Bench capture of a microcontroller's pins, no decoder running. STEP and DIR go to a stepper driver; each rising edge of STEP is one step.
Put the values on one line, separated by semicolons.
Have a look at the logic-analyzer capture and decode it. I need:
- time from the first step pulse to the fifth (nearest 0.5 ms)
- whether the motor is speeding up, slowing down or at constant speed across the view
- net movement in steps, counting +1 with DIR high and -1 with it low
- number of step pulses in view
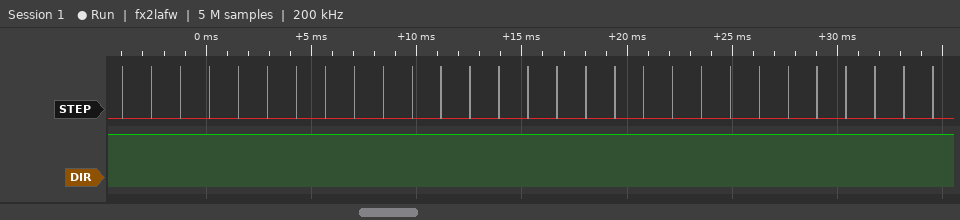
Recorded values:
5.5 ms; constant speed; +29; 29
